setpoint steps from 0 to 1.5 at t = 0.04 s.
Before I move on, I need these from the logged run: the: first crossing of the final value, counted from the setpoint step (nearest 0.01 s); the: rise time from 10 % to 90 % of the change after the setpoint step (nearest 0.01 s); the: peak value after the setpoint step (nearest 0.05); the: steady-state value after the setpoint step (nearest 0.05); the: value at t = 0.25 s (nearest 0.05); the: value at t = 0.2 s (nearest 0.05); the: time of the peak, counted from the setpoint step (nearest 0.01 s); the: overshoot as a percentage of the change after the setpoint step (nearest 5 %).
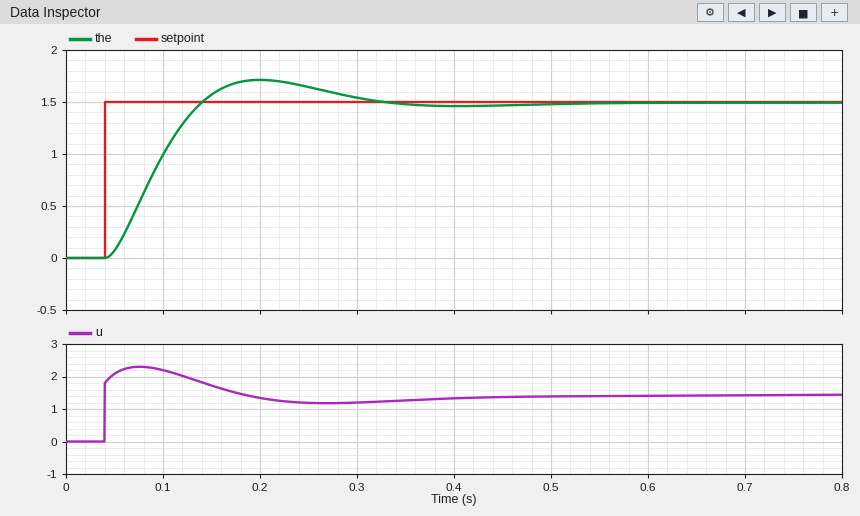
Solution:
0.10 s
0.07 s
1.70
1.50
1.65
1.70
0.16 s
15 %
